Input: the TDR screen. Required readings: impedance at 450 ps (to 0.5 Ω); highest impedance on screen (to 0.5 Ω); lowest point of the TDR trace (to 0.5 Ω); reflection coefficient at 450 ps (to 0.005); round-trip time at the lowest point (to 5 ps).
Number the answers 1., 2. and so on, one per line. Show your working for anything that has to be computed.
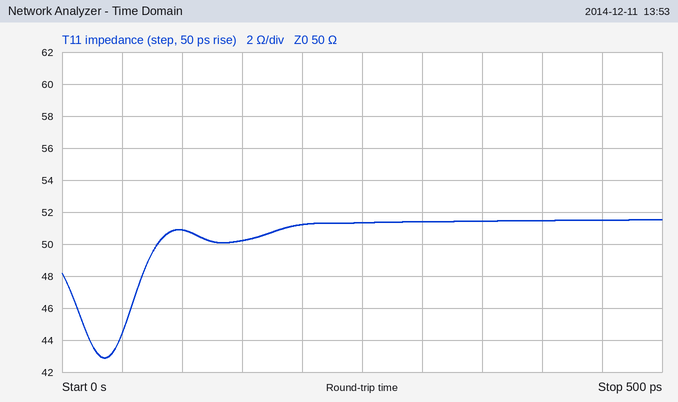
1. 51.5 Ω
2. 51.5 Ω
3. 43.0 Ω
4. (51.5 − 50)/(51.5 + 50) ≈ +0.015
5. 35 ps
